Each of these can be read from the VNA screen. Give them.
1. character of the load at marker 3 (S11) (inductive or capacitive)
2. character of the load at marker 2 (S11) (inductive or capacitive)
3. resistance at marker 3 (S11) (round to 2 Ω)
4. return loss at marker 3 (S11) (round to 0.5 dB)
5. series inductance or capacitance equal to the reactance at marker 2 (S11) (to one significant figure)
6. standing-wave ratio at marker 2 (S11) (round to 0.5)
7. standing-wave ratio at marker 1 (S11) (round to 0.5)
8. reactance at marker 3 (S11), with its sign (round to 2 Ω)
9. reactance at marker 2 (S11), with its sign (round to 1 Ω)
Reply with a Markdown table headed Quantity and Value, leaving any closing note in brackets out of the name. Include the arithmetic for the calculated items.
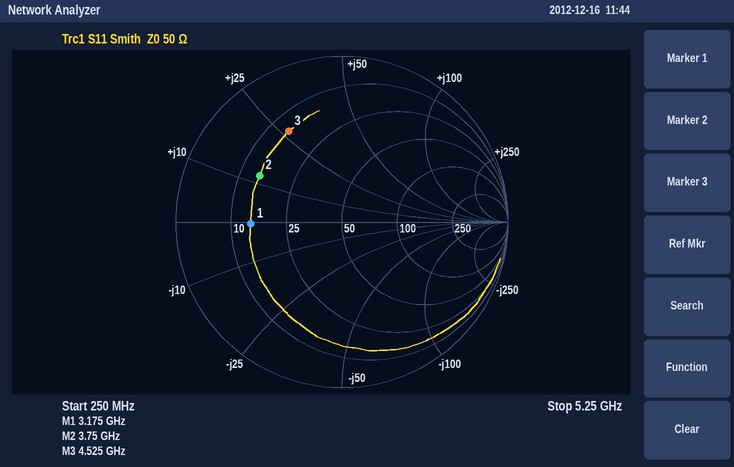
| Quantity | Value |
|---|---|
| character of the load at marker 3 (S11) | inductive |
| character of the load at marker 2 (S11) | inductive |
| resistance at marker 3 (S11) | 14 Ω |
| return loss at marker 3 (S11) | 4.0 dB |
| series inductance or capacitance equal to the reactance at marker 2 (S11) | L = 12 Ω/(2π × 3.75 GHz) ≈ 509 pH, so 500 pH to one significant figure |
| standing-wave ratio at marker 2 (S11) | 3.5 |
| standing-wave ratio at marker 1 (S11) | 3.5 |
| reactance at marker 3 (S11), with its sign | +26 Ω |
| reactance at marker 2 (S11), with its sign | +12 Ω |
